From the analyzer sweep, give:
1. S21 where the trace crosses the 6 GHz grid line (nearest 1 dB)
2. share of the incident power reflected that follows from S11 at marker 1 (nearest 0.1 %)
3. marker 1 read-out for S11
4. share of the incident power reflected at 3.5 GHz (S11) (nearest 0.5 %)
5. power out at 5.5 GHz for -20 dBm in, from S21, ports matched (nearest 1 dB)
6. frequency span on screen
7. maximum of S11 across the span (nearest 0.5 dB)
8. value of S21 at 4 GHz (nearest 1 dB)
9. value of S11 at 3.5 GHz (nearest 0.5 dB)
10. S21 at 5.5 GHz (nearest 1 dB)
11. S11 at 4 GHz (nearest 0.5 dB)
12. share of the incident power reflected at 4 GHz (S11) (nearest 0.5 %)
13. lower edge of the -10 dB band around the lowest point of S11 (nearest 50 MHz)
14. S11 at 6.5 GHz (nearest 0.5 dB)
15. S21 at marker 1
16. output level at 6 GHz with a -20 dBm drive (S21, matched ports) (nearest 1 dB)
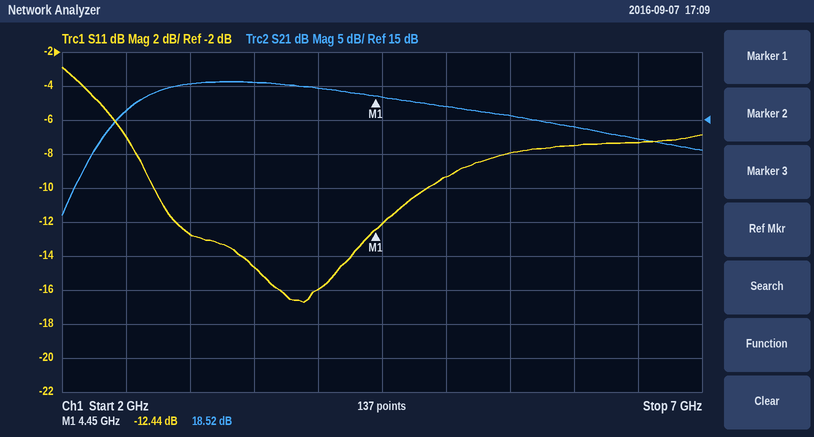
14 dB
5.7 %
-12.44 dB
3.5 %
-4 dBm
5 GHz
-3.0 dB
20 dB
-14.5 dB
16 dB
-16.0 dB
2.5 %
2.70 GHz
-7.5 dB
18.52 dB
-6 dBm
